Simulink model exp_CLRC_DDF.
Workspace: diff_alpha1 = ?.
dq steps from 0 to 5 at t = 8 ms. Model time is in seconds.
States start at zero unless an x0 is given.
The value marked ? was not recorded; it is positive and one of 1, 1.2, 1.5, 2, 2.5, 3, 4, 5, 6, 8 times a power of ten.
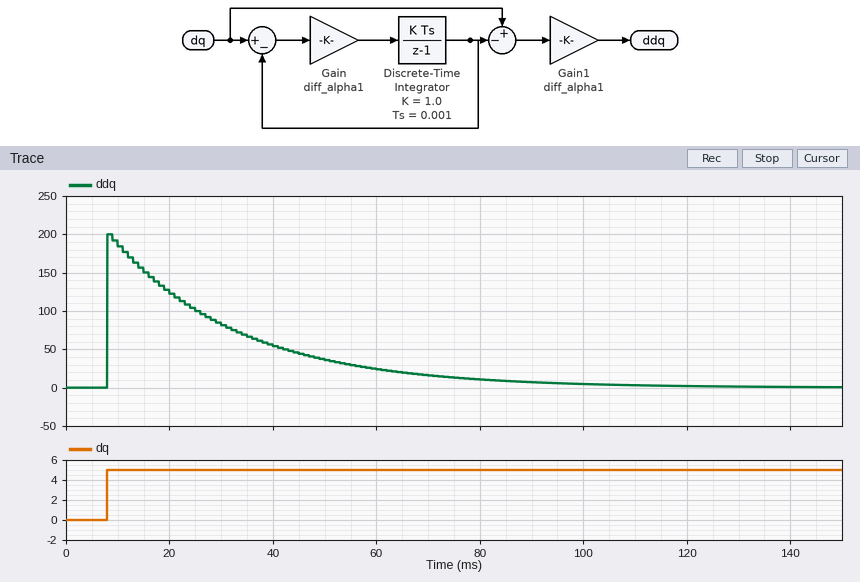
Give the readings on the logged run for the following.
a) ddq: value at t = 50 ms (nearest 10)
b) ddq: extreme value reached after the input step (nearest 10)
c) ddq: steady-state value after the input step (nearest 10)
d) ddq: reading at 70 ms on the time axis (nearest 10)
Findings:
40
200
0
20
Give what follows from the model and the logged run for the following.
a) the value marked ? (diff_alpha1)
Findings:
40
